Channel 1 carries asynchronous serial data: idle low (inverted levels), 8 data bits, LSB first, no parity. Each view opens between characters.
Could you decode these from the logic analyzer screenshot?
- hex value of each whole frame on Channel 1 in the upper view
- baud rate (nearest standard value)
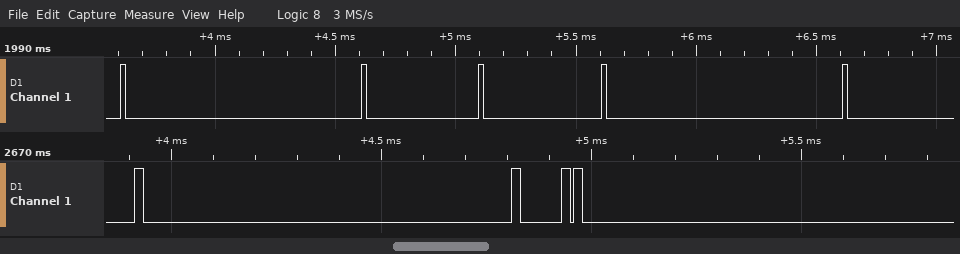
FF, FF, FF, FF, FF
38400 baud
